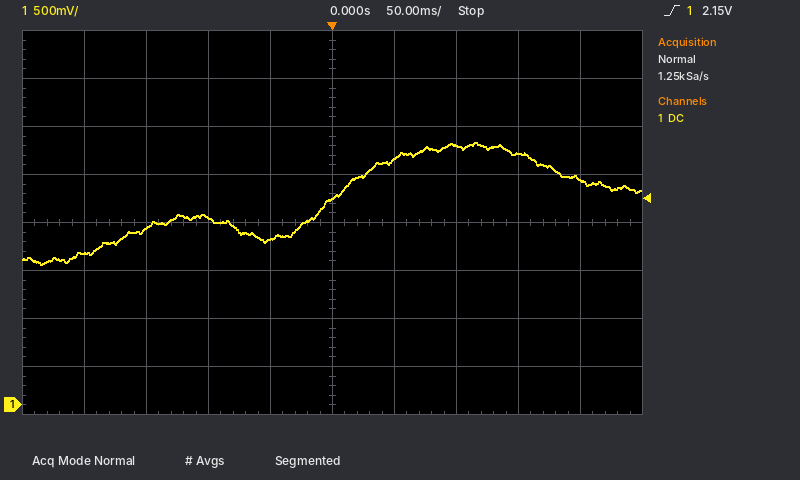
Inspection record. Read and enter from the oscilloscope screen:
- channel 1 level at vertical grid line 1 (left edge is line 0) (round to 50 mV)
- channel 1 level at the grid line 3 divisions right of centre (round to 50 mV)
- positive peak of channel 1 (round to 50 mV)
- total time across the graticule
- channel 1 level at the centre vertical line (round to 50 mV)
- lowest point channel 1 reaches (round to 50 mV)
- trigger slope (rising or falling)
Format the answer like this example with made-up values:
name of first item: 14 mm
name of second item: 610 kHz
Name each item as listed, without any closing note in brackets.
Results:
channel 1 level at vertical grid line 1 (left edge is line 0): 1.60 V
channel 1 level at the grid line 3 divisions right of centre: 2.60 V
positive peak of channel 1: 2.75 V
total time across the graticule: 500 ms
channel 1 level at the centre vertical line: 2.15 V
lowest point channel 1 reaches: 1.45 V
trigger slope: rising
